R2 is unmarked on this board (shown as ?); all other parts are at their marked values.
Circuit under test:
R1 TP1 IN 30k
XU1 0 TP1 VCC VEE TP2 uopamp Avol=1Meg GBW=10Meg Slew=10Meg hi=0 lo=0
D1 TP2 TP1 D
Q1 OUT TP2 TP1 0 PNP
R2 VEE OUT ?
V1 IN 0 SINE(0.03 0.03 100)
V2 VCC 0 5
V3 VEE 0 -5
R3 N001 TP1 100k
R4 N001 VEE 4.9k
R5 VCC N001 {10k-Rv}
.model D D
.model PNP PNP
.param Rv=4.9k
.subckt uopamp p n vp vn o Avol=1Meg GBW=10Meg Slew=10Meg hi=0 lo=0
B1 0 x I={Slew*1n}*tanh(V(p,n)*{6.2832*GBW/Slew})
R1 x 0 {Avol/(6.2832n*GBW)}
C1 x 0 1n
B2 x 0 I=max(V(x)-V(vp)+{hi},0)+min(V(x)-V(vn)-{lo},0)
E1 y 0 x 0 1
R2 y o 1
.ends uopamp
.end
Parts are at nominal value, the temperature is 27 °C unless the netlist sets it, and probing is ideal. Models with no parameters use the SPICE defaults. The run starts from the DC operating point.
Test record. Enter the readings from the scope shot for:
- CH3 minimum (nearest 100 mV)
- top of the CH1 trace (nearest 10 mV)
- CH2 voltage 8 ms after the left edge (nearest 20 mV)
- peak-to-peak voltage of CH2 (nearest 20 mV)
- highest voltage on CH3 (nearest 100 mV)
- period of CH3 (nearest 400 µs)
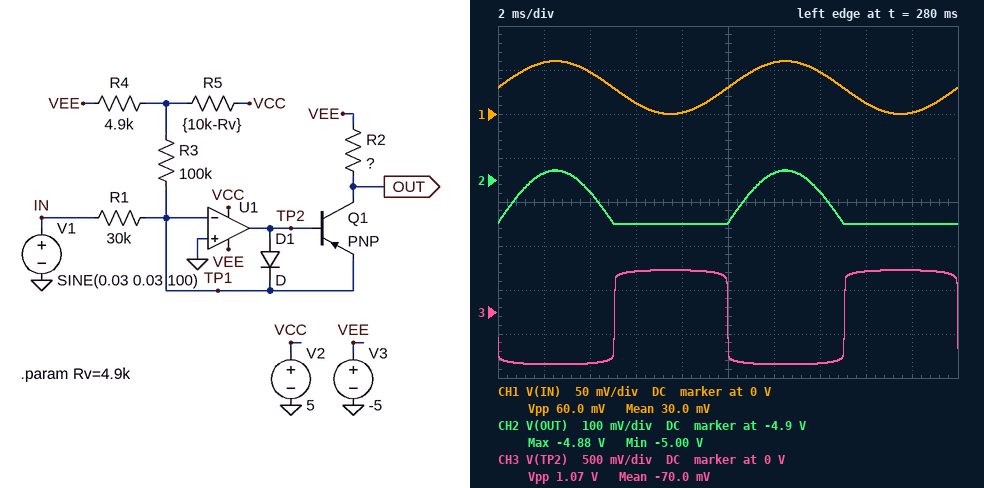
-600 mV
60 mV
-5.00 V
120 mV
500 mV
10.0 ms
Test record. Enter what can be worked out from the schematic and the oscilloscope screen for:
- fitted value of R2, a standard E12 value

120 kΩ
